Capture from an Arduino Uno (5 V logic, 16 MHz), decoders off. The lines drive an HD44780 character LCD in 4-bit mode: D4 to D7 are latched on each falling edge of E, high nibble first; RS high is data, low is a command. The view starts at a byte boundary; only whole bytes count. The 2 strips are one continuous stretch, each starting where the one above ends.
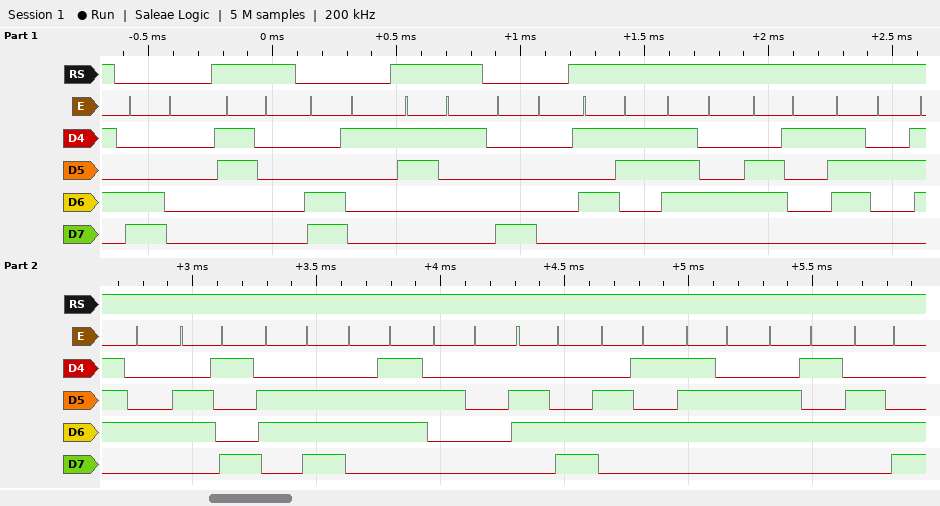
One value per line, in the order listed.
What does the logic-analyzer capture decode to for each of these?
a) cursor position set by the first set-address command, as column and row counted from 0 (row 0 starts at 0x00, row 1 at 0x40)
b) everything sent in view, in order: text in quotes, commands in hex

column 0, row 1
0xC0 "0" 0xC1 "1" 0x80 "Starting level"
